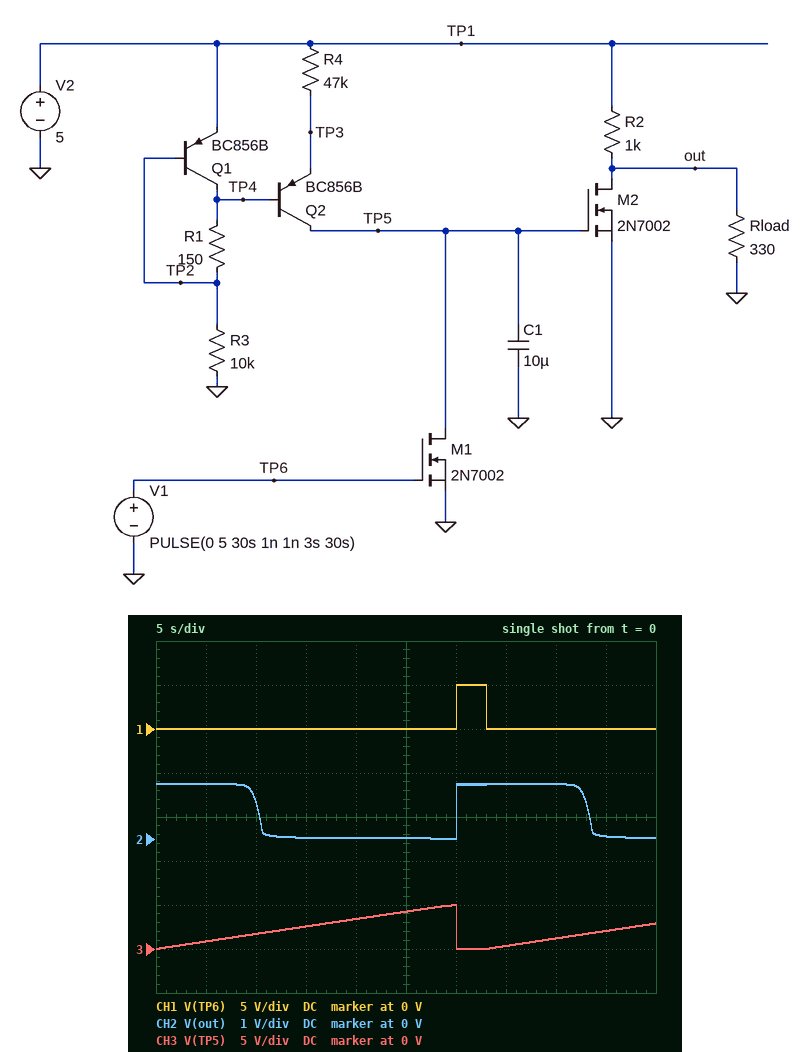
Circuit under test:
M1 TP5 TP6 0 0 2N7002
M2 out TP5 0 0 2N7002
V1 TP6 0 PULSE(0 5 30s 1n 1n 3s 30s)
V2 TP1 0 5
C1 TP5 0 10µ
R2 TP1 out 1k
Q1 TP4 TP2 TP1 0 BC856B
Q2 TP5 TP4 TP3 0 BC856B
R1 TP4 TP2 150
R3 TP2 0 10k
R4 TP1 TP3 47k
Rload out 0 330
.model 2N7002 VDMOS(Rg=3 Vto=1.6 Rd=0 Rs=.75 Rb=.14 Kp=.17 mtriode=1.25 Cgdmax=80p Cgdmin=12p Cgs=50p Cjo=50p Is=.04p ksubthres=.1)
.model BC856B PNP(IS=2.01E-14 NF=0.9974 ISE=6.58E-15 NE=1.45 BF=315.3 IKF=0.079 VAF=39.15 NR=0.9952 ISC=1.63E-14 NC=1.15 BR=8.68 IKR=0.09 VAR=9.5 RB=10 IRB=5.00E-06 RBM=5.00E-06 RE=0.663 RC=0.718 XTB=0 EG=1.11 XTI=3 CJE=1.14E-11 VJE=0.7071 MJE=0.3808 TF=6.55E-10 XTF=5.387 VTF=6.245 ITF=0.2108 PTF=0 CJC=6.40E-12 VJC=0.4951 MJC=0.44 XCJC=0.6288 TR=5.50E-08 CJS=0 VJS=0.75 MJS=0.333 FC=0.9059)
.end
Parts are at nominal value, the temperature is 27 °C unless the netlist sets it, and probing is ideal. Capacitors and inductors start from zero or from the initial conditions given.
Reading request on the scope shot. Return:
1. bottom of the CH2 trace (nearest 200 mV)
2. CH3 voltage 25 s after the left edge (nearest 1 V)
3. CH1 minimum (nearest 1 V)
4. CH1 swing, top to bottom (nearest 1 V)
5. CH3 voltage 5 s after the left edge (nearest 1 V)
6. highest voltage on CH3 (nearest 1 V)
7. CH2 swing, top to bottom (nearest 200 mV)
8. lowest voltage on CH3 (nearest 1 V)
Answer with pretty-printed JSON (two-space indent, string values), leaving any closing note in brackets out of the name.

{
  "bottom of the CH2 trace": "0 V",
  "CH3 voltage 25 s after the left edge": "4 V",
  "CH1 minimum": "0 V",
  "CH1 swing, top to bottom": "5 V",
  "CH3 voltage 5 s after the left edge": "1 V",
  "highest voltage on CH3": "5 V",
  "CH2 swing, top to bottom": "1.2 V",
  "lowest voltage on CH3": "0 V"
}
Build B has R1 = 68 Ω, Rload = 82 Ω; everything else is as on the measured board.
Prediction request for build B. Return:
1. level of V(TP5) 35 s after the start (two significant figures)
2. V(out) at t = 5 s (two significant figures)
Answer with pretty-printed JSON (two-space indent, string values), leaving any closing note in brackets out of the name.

{
  "level of V(TP5) 35 s after the start": "460 mV",
  "V(out) at t = 5 s": "380 mV"
}
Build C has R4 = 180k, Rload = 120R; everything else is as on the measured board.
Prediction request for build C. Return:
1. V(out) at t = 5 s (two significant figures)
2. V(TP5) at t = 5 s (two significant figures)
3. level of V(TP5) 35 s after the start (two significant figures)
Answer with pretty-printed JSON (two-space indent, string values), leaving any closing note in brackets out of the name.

{
  "V(out) at t = 5 s": "540 mV",
  "V(TP5) at t = 5 s": "300 mV",
  "level of V(TP5) 35 s after the start": "120 mV"
}
